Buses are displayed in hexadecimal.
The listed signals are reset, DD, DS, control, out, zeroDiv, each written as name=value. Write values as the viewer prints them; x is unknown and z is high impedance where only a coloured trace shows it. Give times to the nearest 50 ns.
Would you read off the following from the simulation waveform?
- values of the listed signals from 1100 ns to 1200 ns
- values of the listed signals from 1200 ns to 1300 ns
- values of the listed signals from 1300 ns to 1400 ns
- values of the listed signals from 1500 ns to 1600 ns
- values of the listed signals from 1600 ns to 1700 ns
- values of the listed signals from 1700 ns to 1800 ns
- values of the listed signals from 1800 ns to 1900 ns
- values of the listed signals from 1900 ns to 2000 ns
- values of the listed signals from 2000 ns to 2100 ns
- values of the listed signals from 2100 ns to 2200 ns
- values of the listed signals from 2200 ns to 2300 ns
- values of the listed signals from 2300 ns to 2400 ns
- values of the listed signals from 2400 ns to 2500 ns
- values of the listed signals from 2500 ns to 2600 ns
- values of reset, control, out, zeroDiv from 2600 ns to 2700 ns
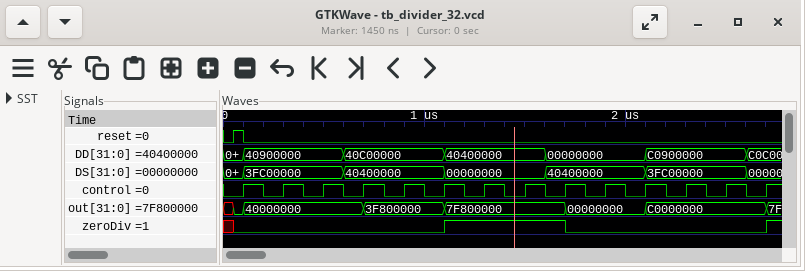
reset=0, DD=40400000, DS=00000000, control=1, out=7F800000, zeroDiv=1
reset=0, DD=40400000, DS=00000000, control=0, out=7F800000, zeroDiv=1
reset=0, DD=40400000, DS=00000000, control=1, out=7F800000, zeroDiv=1
reset=0, DD=40400000, DS=00000000, control=1, out=7F800000, zeroDiv=1
reset=0, DD=00000000, DS=40400000, control=0, out=7F800000, zeroDiv=1
reset=0, DD=00000000, DS=40400000, control=1, out=00000000, zeroDiv=0
reset=0, DD=00000000, DS=40400000, control=0, out=00000000, zeroDiv=0
reset=0, DD=00000000, DS=40400000, control=1, out=00000000, zeroDiv=0
reset=0, DD=00000000, DS=40400000, control=0, out=00000000, zeroDiv=0
reset=0, DD=C0900000, DS=3FC00000, control=1, out=C0000000, zeroDiv=0
reset=0, DD=C0900000, DS=3FC00000, control=0, out=C0000000, zeroDiv=0
reset=0, DD=C0900000, DS=3FC00000, control=1, out=C0000000, zeroDiv=0
reset=0, DD=C0900000, DS=3FC00000, control=0, out=C0000000, zeroDiv=0
reset=0, DD=C0900000, DS=3FC00000, control=1, out=C0000000, zeroDiv=0
reset=0, control=0, out=C0000000, zeroDiv=0
